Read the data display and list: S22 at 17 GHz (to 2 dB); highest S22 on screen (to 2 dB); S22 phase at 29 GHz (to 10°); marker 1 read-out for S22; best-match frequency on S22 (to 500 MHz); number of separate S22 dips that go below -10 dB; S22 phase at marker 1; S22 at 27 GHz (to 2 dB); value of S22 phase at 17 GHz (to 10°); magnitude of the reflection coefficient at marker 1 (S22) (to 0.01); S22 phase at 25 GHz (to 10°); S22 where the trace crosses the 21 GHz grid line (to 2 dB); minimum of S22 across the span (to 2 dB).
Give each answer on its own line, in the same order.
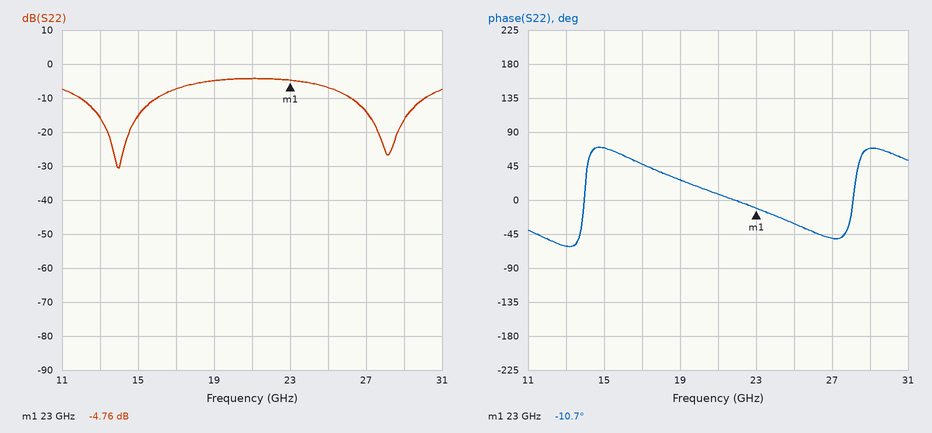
-8 dB
-4 dB
70°
-4.76 dB
14.0 GHz
2
-10.7°
-14 dB
50°
0.58
-30°
-4 dB
-30 dB
